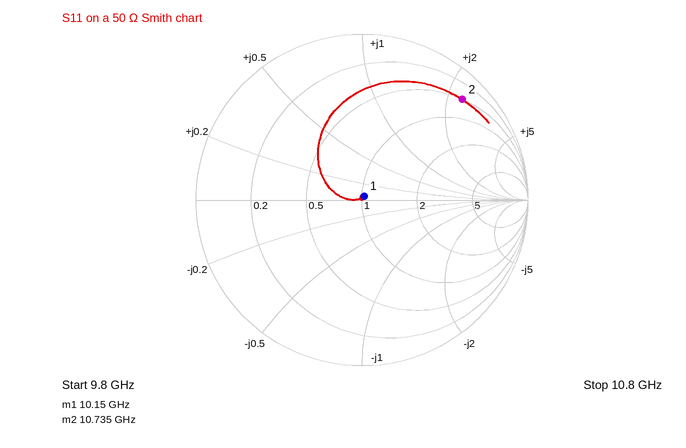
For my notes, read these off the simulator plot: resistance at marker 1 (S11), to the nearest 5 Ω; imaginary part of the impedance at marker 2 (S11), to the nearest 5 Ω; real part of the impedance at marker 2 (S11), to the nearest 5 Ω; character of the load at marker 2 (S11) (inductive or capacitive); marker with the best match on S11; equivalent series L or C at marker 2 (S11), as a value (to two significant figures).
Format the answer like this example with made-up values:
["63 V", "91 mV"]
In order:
["50 Ω", "+115 Ω", "25 Ω", "inductive", "marker 1", "1.7 nH"]
